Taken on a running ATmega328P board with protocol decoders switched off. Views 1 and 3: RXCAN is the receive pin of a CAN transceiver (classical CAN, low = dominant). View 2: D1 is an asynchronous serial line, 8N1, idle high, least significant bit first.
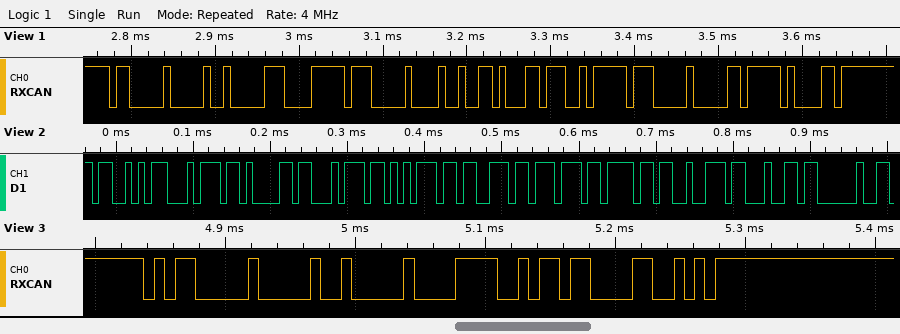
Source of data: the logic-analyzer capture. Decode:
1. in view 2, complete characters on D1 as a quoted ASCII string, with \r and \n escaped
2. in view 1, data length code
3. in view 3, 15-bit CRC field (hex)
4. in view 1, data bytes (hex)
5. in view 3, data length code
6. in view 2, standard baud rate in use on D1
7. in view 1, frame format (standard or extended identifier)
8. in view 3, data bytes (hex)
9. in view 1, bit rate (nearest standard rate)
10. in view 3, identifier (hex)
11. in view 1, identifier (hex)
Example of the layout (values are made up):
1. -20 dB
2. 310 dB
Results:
1. "Statusword "
2. 8
3. 0x6C32
4. 30 FF 00 49 A3 72 FF 00
5. 2
6. 115200 baud
7. standard
8. 00 F2
9. 125 kbit/s
10. 0x580
11. 0x600
